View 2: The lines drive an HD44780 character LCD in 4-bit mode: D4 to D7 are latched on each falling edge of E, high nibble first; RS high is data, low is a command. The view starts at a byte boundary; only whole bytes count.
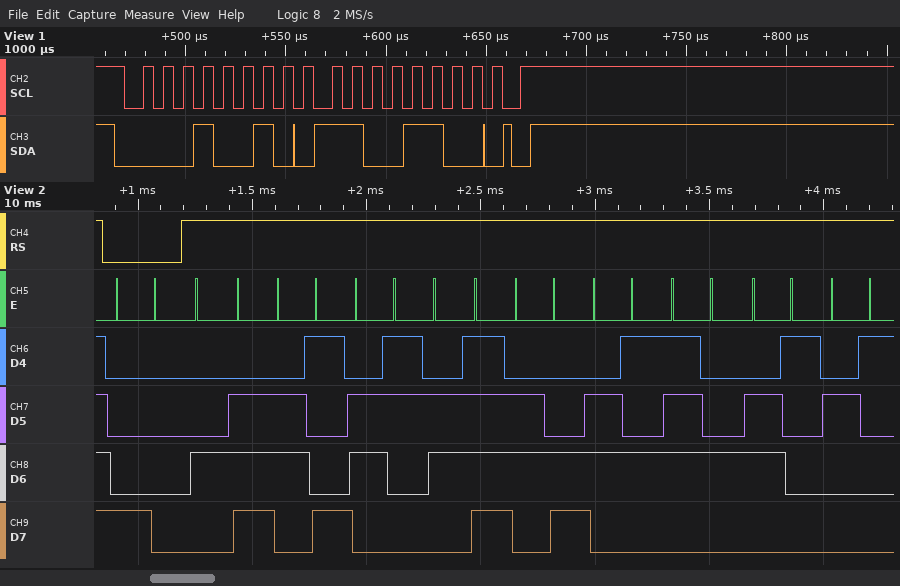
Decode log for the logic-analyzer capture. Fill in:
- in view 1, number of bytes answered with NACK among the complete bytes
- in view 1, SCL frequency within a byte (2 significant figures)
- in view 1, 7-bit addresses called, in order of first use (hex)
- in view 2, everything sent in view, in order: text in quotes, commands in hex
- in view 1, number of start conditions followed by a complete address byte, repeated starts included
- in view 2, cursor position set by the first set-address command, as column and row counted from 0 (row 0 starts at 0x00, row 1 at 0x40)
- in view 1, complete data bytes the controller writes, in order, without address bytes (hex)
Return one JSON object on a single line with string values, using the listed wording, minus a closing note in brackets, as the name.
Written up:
{"in view 1, number of bytes answered with NACK among the complete bytes": "0", "in view 1, SCL frequency within a byte": "100 kHz", "in view 1, 7-bit addresses called, in order of first use": "0x09", "in view 2, everything sent in view, in order: text in quotes, commands in hex": "0x80 \"Nicoleta!\"", "in view 1, number of start conditions followed by a complete address byte, repeated starts included": "1", "in view 2, cursor position set by the first set-address command, as column and row counted from 0": "column 0, row 0", "in view 1, complete data bytes the controller writes, in order, without address bytes": "CC"}
